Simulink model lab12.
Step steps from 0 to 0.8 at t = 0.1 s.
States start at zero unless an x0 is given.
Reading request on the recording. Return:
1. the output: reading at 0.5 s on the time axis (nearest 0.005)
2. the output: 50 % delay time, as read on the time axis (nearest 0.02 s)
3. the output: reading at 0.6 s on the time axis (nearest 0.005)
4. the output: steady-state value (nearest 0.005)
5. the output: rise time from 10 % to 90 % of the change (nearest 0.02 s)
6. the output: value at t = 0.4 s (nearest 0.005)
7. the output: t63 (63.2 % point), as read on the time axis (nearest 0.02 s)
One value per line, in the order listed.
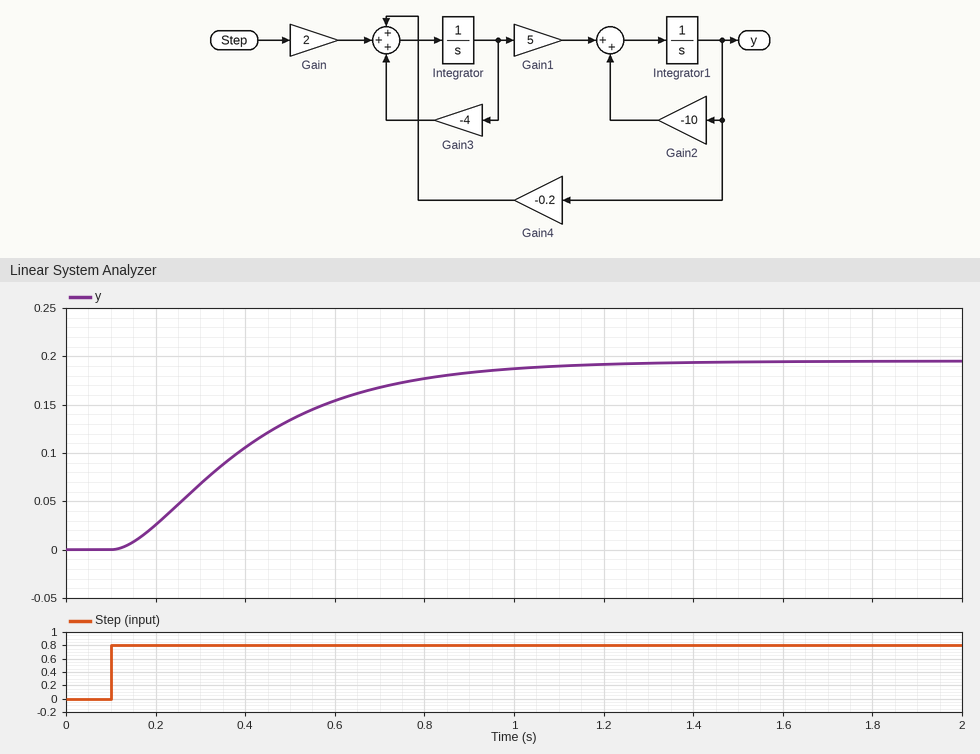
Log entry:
0.135
0.38 s
0.155
0.195
0.60 s
0.105
0.46 s
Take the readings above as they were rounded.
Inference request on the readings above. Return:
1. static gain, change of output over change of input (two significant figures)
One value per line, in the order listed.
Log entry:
0.24
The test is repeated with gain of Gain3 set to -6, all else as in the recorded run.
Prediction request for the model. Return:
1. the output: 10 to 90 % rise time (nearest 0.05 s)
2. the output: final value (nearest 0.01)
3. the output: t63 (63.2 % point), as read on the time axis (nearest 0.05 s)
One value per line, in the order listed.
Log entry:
0.45 s
0.13
0.40 s
